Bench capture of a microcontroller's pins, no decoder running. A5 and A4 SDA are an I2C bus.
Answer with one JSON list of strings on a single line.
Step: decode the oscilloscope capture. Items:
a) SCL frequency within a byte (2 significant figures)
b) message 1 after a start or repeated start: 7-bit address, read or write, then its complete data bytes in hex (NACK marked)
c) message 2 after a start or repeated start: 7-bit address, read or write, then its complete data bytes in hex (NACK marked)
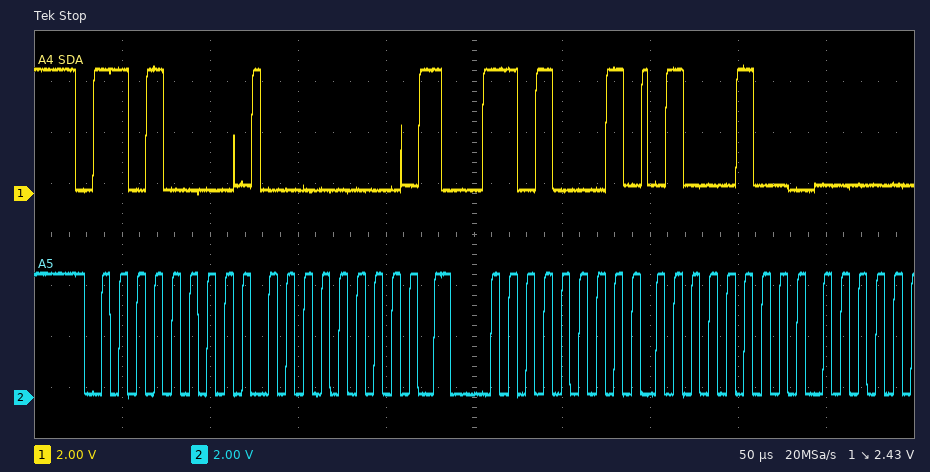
["100 kHz", "0x68 write: 00", "0x68 read: 44"]
